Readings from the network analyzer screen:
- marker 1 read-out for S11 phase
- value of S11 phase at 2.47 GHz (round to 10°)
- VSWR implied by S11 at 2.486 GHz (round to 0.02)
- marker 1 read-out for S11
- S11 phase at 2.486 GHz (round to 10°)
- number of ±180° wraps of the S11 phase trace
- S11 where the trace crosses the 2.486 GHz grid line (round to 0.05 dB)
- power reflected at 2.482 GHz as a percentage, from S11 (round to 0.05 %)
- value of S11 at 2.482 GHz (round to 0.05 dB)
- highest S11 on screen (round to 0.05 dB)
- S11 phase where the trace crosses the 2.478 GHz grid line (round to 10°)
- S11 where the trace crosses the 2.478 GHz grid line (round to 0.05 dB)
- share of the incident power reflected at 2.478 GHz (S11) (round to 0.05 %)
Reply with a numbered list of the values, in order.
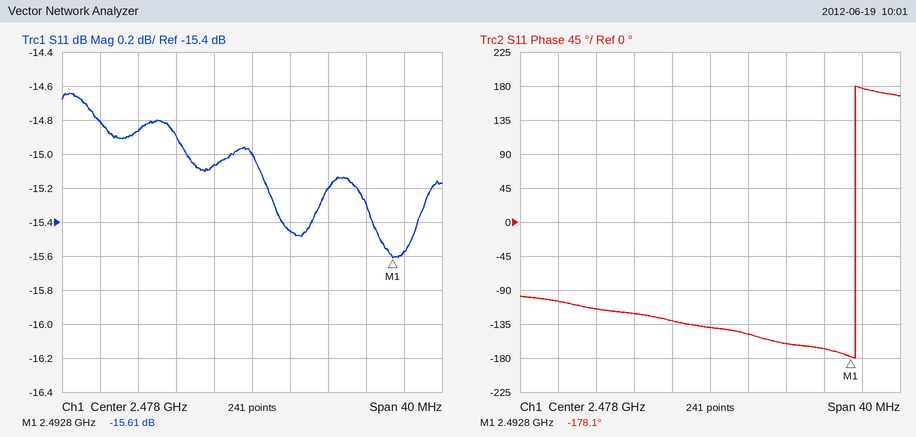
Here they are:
1. -178.1°
2. -120°
3. 1.42
4. -15.61 dB
5. -160°
6. 1
7. -15.20 dB
8. 2.85 %
9. -15.45 dB
10. -14.65 dB
11. -140°
12. -15.00 dB
13. 3.15 %
